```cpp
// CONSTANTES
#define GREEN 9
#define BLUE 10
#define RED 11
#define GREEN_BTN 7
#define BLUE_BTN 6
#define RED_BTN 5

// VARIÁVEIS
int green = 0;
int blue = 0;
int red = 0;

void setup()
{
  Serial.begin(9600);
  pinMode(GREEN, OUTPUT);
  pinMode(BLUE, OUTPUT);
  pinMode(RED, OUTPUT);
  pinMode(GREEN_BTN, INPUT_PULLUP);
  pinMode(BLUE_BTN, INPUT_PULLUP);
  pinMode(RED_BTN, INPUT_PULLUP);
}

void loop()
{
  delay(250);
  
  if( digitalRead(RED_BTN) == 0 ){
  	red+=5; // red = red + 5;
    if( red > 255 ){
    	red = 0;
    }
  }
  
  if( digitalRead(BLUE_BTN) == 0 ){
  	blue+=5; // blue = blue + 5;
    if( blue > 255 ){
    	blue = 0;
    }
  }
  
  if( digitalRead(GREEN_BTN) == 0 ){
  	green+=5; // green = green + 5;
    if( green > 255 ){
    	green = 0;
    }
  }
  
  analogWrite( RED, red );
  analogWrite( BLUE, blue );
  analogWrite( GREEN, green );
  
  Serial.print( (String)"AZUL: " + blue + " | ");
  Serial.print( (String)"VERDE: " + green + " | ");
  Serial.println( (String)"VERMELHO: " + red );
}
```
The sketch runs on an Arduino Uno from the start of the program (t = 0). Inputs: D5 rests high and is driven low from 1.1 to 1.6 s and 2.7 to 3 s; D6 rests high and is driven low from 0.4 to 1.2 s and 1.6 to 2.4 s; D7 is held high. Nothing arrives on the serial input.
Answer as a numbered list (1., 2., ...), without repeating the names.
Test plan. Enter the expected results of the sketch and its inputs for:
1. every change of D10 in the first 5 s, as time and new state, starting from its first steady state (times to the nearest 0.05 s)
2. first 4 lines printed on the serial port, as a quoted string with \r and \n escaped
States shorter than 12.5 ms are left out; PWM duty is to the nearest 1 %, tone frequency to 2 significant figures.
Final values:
1. 0 s low; 0.5 s PWM 2 %; 0.75 s PWM 4 %; 1 s PWM 6 %; 1.75 s PWM 8 %; 2 s PWM 10 %; 2.25 s PWM 12 %
2. "AZUL: 0 | VERDE: 0 | VERMELHO: 0\r\nAZUL: 5 | VERDE: 0 | VERMELHO: 0\r\nAZUL: 10 | VERDE: 0 | VERMELHO: 0\r\nAZUL: 15 | VERDE: 0 | VERMELHO: 0\r\n"
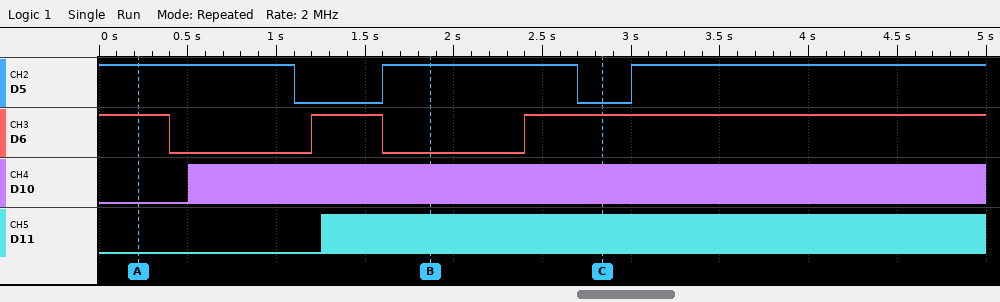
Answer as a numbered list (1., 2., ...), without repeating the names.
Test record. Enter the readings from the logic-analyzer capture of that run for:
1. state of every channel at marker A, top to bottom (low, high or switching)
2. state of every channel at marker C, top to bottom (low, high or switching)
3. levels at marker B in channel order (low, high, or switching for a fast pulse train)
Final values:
1. D5 high, D6 high, D10 low, D11 low
2. D5 low, D6 high, D10 switching, D11 switching
3. D5 high, D6 low, D10 switching, D11 switching
